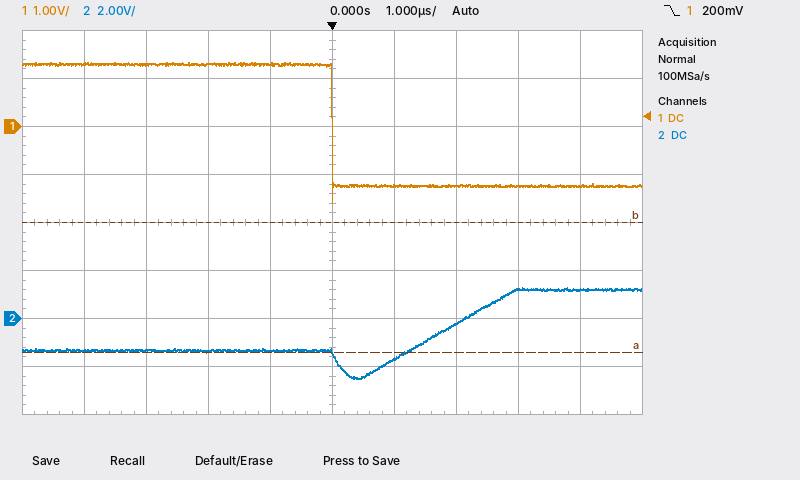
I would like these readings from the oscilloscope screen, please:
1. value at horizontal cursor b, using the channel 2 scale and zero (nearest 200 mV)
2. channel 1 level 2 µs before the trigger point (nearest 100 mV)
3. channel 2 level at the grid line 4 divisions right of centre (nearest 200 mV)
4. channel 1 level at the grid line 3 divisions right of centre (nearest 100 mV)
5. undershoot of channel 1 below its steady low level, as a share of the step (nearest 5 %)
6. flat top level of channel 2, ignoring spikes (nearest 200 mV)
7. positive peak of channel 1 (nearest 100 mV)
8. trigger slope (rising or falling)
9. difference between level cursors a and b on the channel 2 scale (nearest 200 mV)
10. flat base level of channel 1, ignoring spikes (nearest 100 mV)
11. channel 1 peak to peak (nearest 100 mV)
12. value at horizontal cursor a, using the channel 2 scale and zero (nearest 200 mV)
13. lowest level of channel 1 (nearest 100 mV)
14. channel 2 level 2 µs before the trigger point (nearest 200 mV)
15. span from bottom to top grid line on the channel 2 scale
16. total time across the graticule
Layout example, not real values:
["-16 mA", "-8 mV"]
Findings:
["4.0 V", "1.3 V", "1.2 V", "-1.2 V", "15 %", "1.2 V", "1.3 V", "falling", "5.4 V", "-1.2 V", "2.9 V", "-1.4 V", "-1.6 V", "-1.4 V", "16 V", "10 µs"]
